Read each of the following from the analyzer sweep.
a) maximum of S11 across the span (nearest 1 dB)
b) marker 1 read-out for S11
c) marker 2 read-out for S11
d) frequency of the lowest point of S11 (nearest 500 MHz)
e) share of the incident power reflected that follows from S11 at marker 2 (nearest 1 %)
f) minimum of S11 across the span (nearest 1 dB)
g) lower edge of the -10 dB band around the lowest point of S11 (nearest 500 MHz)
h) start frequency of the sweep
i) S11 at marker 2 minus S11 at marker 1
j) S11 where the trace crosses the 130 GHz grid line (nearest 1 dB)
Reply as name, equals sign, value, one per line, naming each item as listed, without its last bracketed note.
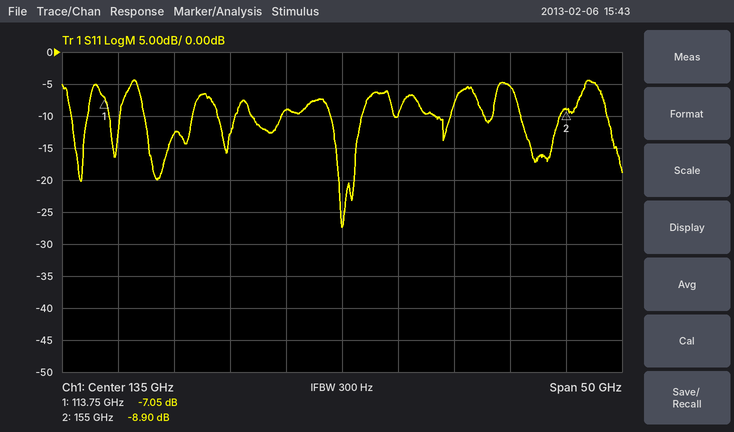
maximum of S11 across the span = -4 dB
marker 1 read-out for S11 = -7.05 dB
marker 2 read-out for S11 = -8.90 dB
frequency of the lowest point of S11 = 135.0 GHz
share of the incident power reflected that follows from S11 at marker 2 = 13 %
minimum of S11 across the span = -27 dB
lower edge of the -10 dB band around the lowest point of S11 = 134.0 GHz
start frequency of the sweep = 110 GHz
S11 at marker 2 minus S11 at marker 1 = -1.85 dB
S11 where the trace crosses the 130 GHz grid line = -9 dB
